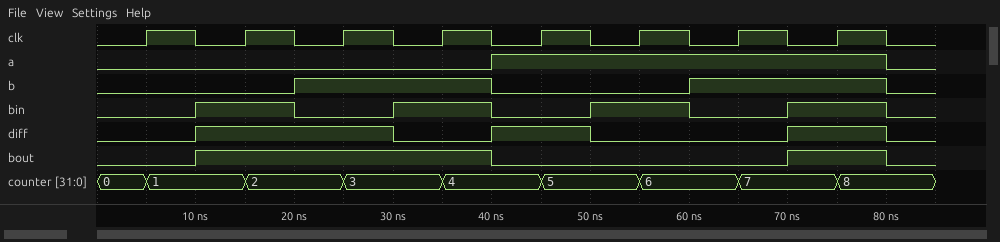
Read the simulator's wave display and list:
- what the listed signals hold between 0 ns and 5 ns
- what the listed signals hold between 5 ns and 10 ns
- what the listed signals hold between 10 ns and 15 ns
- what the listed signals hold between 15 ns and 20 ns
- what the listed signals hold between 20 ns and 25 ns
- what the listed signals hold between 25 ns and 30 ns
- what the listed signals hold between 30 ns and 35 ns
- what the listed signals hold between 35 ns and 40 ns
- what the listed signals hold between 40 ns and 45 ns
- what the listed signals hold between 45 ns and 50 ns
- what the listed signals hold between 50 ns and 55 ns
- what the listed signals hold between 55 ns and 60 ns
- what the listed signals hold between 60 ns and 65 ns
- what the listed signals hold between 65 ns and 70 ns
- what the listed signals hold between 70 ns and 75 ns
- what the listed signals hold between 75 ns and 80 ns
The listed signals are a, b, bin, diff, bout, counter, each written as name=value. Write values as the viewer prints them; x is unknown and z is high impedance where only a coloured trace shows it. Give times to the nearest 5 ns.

a=0, b=0, bin=0, diff=0, bout=0, counter=0
a=0, b=0, bin=0, diff=0, bout=0, counter=1
a=0, b=0, bin=1, diff=1, bout=1, counter=1
a=0, b=0, bin=1, diff=1, bout=1, counter=2
a=0, b=1, bin=0, diff=1, bout=1, counter=2
a=0, b=1, bin=0, diff=1, bout=1, counter=3
a=0, b=1, bin=1, diff=0, bout=1, counter=3
a=0, b=1, bin=1, diff=0, bout=1, counter=4
a=1, b=0, bin=0, diff=1, bout=0, counter=4
a=1, b=0, bin=0, diff=1, bout=0, counter=5
a=1, b=0, bin=1, diff=0, bout=0, counter=5
a=1, b=0, bin=1, diff=0, bout=0, counter=6
a=1, b=1, bin=0, diff=0, bout=0, counter=6
a=1, b=1, bin=0, diff=0, bout=0, counter=7
a=1, b=1, bin=1, diff=1, bout=1, counter=7
a=1, b=1, bin=1, diff=1, bout=1, counter=8
